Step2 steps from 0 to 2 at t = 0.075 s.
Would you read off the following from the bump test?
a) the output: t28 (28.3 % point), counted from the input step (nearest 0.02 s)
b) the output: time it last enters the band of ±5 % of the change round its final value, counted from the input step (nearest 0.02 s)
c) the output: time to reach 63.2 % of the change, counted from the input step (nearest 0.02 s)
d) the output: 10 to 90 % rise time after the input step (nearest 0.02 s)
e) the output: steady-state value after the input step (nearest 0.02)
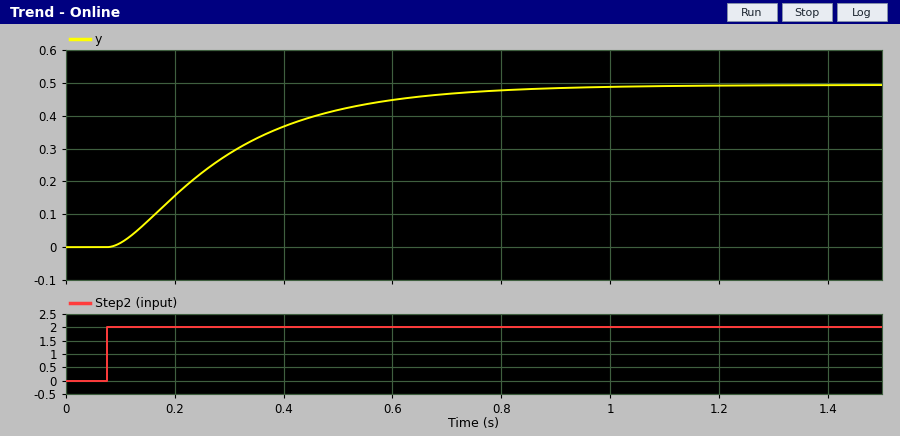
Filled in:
0.12 s
0.64 s
0.26 s
0.46 s
0.50
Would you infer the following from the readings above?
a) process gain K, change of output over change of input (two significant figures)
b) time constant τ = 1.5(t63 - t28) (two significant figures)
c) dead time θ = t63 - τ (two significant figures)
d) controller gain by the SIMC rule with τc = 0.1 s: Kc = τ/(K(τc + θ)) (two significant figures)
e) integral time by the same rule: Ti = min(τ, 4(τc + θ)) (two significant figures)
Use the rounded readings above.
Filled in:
0.25
0.21 s
0.050 s
5.6
0.21 s
